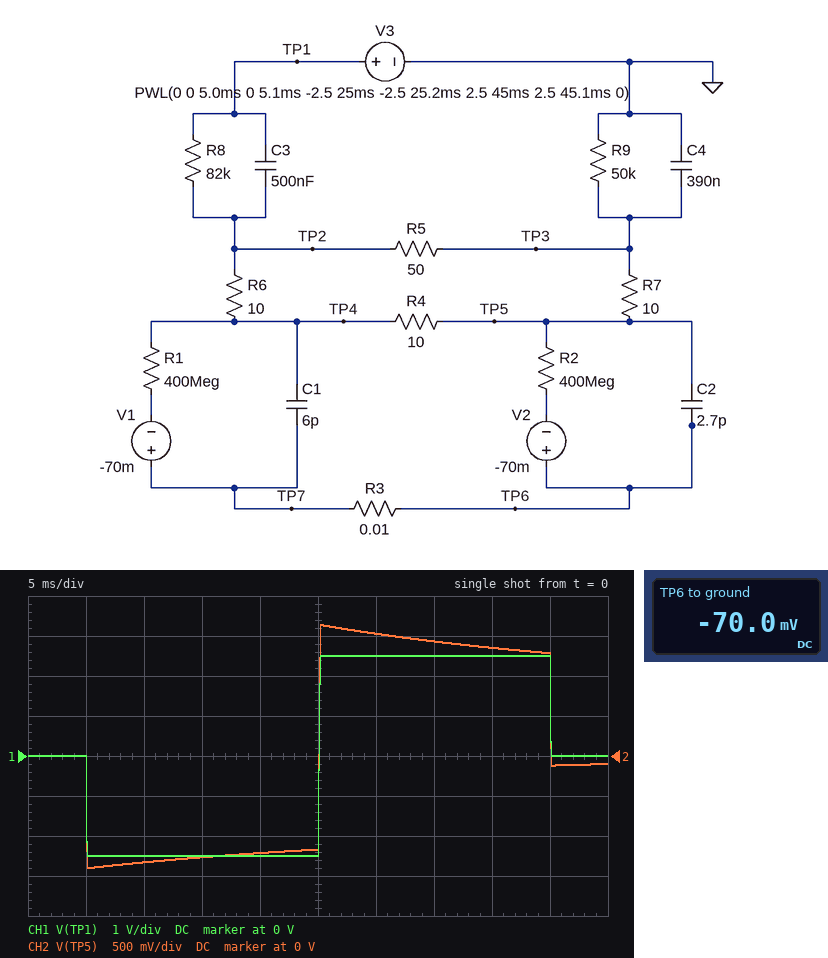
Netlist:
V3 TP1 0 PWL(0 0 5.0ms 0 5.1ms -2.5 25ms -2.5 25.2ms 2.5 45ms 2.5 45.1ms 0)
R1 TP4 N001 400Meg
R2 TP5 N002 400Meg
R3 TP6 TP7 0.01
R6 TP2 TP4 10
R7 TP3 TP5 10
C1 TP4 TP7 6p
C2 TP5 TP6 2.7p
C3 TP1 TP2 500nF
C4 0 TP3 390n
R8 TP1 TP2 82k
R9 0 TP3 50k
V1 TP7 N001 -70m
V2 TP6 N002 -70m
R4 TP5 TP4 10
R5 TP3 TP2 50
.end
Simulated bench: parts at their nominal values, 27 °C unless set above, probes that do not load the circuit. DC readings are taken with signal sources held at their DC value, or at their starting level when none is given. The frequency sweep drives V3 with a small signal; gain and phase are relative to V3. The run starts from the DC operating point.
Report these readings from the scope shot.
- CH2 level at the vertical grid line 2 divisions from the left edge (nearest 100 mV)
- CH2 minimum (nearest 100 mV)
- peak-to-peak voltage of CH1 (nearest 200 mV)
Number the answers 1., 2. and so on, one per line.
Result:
1. -1.3 V
2. -1.4 V
3. 5.0 V
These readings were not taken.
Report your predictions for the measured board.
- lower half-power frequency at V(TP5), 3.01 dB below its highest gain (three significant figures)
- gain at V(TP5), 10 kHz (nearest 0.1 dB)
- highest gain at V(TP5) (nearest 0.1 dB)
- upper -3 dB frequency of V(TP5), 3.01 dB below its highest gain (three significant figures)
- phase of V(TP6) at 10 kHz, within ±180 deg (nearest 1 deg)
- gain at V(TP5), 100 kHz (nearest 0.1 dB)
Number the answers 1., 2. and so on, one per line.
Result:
1. 1.73 Hz
2. -5.2 dB
3. -5.0 dB
4. 71.3 kHz
5. 0 deg
6. -8.6 dB
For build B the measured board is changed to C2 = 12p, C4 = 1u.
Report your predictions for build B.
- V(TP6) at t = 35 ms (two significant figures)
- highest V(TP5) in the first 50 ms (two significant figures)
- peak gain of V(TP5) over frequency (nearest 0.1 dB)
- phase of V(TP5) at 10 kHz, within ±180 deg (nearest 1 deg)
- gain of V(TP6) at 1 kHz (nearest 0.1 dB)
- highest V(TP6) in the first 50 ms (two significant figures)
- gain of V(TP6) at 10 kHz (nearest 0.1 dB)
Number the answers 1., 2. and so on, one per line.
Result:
1. 750 mV
2. 850 mV
3. -8.4 dB
4. 0 deg
5. -9.5 dB
6. 780 mV
7. -9.1 dB
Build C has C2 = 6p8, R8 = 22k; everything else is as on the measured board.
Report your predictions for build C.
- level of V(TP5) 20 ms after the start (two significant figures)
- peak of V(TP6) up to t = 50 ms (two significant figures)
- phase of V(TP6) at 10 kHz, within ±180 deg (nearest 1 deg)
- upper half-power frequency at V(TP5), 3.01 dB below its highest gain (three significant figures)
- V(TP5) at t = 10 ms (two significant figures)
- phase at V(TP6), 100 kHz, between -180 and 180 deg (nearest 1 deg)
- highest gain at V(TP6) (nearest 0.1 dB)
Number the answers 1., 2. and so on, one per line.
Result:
1. -1.6 V
2. 1.5 V
3. -2 deg
4. 29.3 kHz
5. -1.5 V
6. -3 deg
7. -3.2 dB
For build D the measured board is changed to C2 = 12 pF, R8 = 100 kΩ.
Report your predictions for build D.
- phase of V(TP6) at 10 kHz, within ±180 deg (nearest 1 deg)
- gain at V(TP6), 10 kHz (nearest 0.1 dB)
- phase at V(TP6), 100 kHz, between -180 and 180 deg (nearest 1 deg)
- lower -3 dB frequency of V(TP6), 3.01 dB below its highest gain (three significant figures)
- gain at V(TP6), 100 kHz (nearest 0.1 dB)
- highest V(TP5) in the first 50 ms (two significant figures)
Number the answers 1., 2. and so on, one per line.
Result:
1. -3 deg
2. -5.1 dB
3. -5 deg
4. 2.92 Hz
5. -6.7 dB
6. 1.7 V
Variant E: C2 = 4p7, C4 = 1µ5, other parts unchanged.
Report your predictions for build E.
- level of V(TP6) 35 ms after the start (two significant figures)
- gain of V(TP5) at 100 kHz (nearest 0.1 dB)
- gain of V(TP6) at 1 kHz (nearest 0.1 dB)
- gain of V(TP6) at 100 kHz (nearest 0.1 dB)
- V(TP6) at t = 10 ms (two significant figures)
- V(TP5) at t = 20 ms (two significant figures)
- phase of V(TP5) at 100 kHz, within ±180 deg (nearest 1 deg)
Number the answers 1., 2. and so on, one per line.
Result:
1. 530 mV
2. -9.6 dB
3. -12.0 dB
4. -5.8 dB
5. -720 mV
6. -690 mV
7. 3 deg
